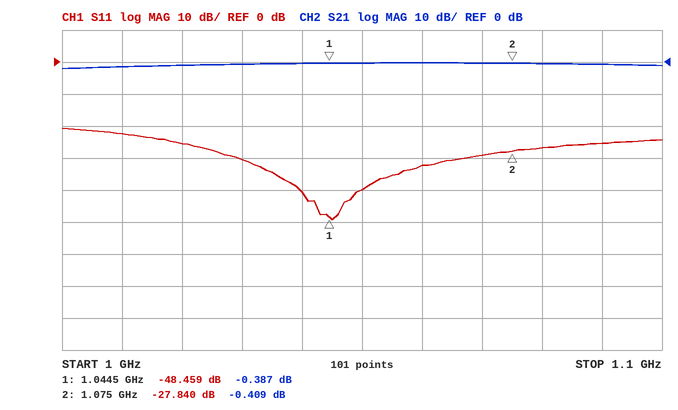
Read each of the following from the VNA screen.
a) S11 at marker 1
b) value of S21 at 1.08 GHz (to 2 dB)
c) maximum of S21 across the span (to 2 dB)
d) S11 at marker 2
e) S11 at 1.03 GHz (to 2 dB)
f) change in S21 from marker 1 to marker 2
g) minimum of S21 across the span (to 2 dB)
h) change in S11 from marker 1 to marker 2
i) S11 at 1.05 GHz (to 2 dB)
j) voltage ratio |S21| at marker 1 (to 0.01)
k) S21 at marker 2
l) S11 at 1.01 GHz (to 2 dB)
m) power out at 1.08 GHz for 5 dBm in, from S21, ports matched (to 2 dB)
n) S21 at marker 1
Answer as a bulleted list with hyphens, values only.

- -48.459 dB
- 0 dB
- 0 dB
- -27.840 dB
- -30 dB
- -0.022 dB
- -2 dB
- 20.619 dB
- -40 dB
- 0.96
- -0.409 dB
- -22 dB
- 4 dBm
- -0.387 dB
